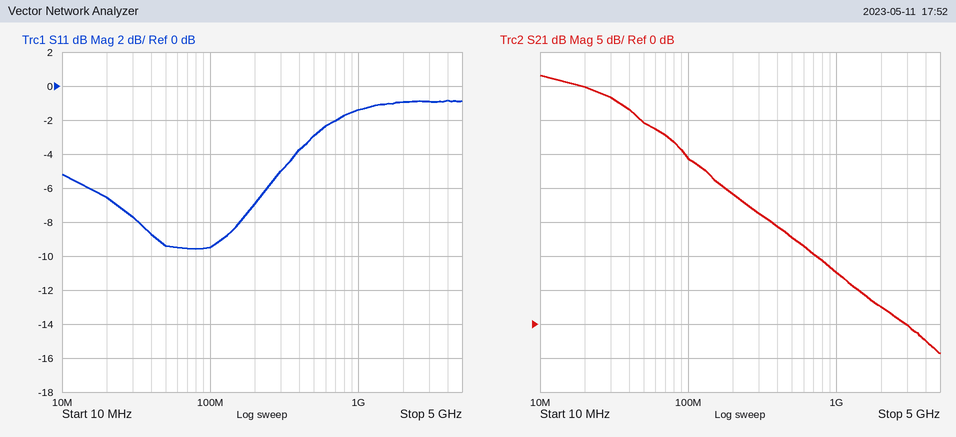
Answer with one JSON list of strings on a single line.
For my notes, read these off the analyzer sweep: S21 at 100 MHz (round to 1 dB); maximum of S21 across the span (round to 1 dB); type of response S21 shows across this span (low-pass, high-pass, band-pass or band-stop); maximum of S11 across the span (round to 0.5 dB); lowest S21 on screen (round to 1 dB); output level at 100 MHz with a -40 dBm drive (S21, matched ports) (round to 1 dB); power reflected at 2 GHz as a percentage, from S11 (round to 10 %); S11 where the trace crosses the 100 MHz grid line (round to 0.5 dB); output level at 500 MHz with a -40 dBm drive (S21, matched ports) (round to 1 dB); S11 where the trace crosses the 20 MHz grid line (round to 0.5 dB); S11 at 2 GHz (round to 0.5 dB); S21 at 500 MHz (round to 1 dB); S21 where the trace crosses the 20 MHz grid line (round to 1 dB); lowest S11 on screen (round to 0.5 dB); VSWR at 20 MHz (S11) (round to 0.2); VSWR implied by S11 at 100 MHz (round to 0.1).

["24 dB", "37 dB", "low-pass", "-1.0 dB", "-4 dB", "-16 dBm", "80 %", "-9.5 dB", "-27 dBm", "-6.5 dB", "-1.0 dB", "13 dB", "35 dB", "-9.5 dB", "2.8", "2.0"]
